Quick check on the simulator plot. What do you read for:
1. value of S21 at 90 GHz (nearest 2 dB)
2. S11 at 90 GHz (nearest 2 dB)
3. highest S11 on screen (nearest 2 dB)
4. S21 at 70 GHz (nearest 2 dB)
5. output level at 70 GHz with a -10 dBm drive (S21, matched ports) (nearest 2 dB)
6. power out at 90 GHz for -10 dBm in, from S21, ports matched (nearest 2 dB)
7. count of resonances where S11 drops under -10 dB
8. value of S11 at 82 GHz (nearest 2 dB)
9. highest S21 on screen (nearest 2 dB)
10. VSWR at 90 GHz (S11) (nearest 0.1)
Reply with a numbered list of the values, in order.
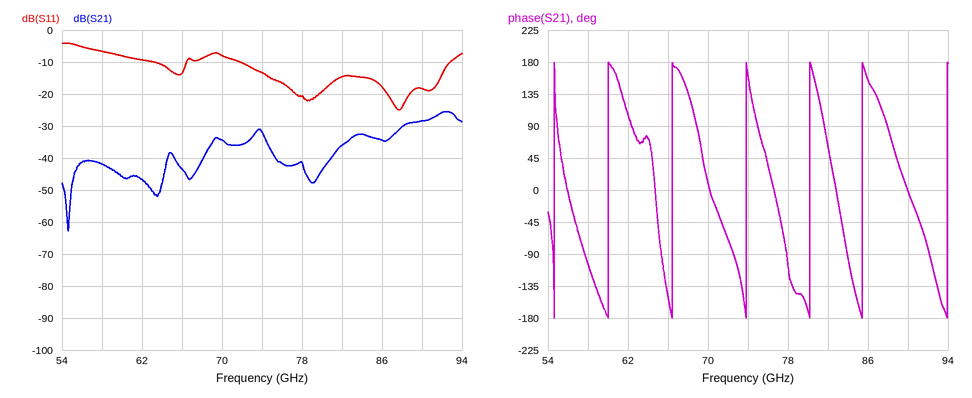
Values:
1. -28 dB
2. -18 dB
3. -4 dB
4. -34 dB
5. -44 dBm
6. -38 dBm
7. 3
8. -14 dB
9. -26 dB
10. 1.3
